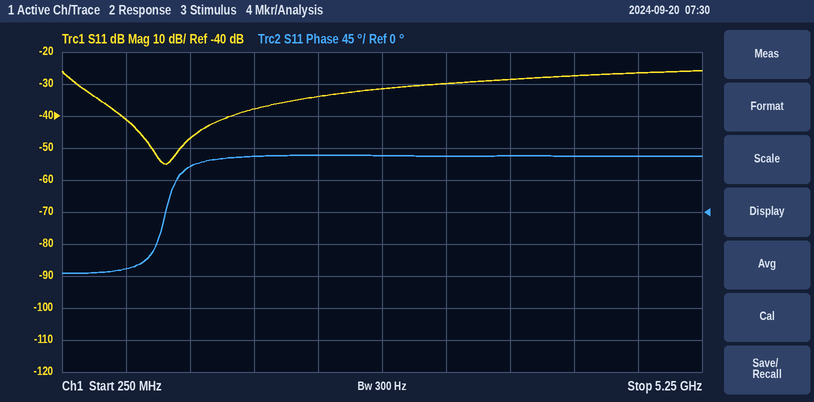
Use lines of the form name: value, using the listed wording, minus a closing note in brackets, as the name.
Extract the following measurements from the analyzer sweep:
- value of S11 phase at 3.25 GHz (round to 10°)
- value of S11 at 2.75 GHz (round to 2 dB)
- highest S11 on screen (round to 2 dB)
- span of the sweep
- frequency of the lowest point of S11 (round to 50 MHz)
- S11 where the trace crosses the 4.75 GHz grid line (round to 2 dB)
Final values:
value of S11 phase at 3.25 GHz: 80°
value of S11 at 2.75 GHz: -32 dB
highest S11 on screen: -26 dB
span of the sweep: 5 GHz
frequency of the lowest point of S11: 1.05 GHz
S11 where the trace crosses the 4.75 GHz grid line: -26 dB
